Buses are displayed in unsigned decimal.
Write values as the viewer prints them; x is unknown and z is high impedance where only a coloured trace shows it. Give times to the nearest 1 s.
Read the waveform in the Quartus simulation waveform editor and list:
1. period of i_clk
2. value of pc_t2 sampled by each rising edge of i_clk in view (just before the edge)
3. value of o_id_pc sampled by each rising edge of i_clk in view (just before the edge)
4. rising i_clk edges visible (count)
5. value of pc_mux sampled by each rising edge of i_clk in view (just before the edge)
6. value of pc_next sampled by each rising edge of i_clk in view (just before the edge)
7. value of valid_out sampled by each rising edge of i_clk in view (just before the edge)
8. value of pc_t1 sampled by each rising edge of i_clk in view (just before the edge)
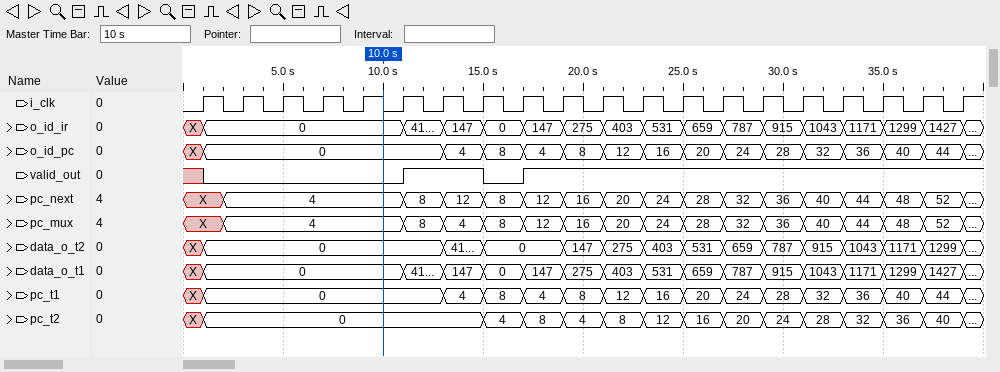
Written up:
2 s
X, 0, 0, 0, 0, 0, 0, 0, 4, 8, 4, 8, 12, 16, 20, 24, 28, 32, 36, 40
X, 0, 0, 0, 0, 0, 0, 4, 8, 4, 8, 12, 16, 20, 24, 28, 32, 36, 40, 44
20
X, 4, 4, 4, 4, 4, 8, 4, 8, 12, 16, 20, 24, 28, 32, 36, 40, 44, 48, 52
X, 4, 4, 4, 4, 4, 8, 12, 8, 12, 16, 20, 24, 28, 32, 36, 40, 44, 48, 52
x 0 0 0 0 0 1 1 0 1 1 1 1 1 1 1 1 1 1 1
X, 0, 0, 0, 0, 0, 0, 4, 8, 4, 8, 12, 16, 20, 24, 28, 32, 36, 40, 44
